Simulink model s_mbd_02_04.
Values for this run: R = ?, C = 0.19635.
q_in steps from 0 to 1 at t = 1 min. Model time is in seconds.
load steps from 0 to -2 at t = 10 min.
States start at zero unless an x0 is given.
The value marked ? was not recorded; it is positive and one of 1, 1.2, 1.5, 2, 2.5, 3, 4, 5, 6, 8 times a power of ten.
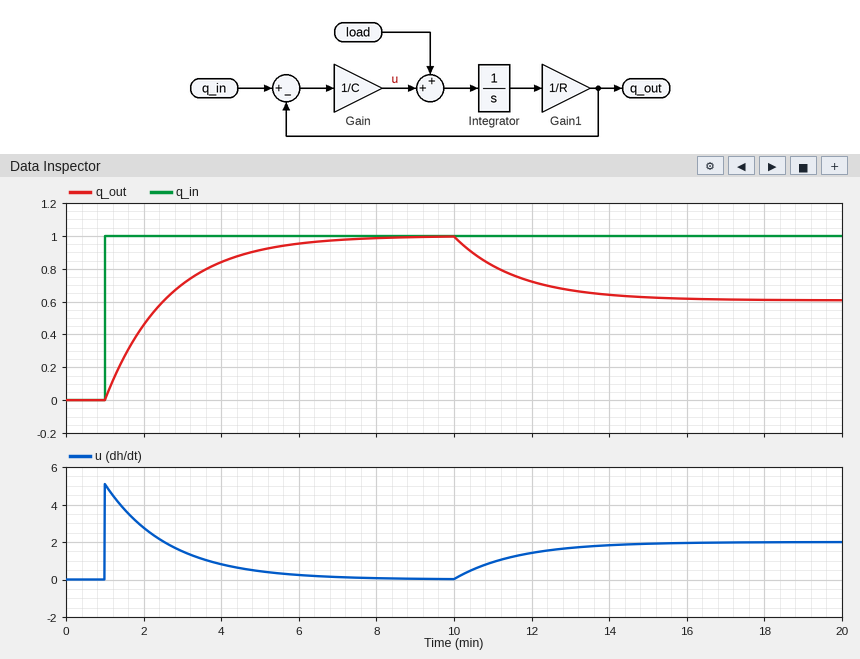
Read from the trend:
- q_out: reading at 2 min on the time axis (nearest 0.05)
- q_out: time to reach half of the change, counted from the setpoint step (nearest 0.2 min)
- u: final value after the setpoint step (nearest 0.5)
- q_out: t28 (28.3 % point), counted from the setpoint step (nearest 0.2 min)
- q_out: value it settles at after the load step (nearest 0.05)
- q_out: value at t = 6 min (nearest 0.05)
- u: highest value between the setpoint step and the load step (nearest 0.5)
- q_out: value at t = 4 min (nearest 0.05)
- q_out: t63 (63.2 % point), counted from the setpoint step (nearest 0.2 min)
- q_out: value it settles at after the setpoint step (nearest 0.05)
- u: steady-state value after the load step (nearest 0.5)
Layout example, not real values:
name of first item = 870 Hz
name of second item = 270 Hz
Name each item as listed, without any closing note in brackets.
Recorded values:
q_out: reading at 2 min on the time axis = 0.45
q_out: time to reach half of the change, counted from the setpoint step = 1.2 min
u: final value after the setpoint step = 0.0
q_out: t28 (28.3 % point), counted from the setpoint step = 0.6 min
q_out: value it settles at after the load step = 0.60
q_out: value at t = 6 min = 0.95
u: highest value between the setpoint step and the load step = 5.0
q_out: value at t = 4 min = 0.85
q_out: t63 (63.2 % point), counted from the setpoint step = 1.6 min
q_out: value it settles at after the setpoint step = 1.00
u: steady-state value after the load step = 2.0
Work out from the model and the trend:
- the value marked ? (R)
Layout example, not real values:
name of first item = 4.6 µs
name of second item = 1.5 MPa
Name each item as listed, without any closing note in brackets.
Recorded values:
the value marked ? = 500
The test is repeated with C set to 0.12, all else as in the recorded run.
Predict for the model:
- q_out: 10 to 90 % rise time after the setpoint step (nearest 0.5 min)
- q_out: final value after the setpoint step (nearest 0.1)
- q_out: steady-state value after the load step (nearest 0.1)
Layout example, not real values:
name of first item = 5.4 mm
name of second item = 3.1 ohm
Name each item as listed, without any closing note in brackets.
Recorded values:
q_out: 10 to 90 % rise time after the setpoint step = 2.0 min
q_out: final value after the setpoint step = 1.0
q_out: steady-state value after the load step = 0.8
